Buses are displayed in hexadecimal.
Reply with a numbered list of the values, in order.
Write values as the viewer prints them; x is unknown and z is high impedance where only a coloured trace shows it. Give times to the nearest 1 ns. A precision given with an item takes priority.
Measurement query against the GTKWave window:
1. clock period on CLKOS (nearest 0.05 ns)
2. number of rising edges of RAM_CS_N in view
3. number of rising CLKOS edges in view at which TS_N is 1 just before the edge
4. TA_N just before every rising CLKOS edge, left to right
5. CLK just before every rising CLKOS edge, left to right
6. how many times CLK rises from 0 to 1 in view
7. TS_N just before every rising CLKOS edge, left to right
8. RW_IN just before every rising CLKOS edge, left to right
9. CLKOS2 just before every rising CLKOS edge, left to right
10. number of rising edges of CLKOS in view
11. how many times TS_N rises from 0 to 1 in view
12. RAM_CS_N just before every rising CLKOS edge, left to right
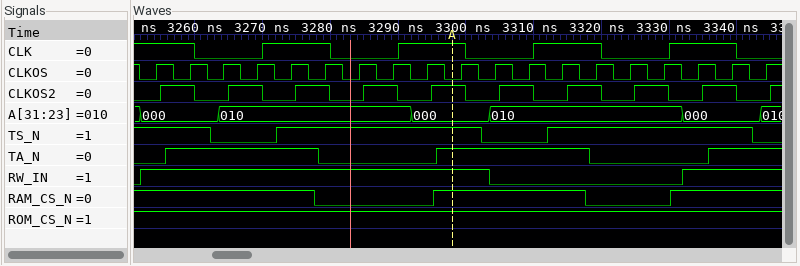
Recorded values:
1. 5 ns
2. 2
3. 14
4. 0 1 1 1 1 0 0 0 0 1 1 1 1 0 0 0 0 1 1
5. 1 1 0 0 1 1 0 0 1 1 0 0 1 1 0 0 1 1 0
6. 4
7. 1 1 0 0 1 1 1 1 1 1 0 0 1 1 1 1 1 1 0
8. 1 1 1 1 1 1 1 1 1 1 0 0 0 0 0 0 1 1 1
9. 0 1 0 1 0 1 0 1 0 1 0 1 0 1 0 1 0 1 0
10. 19
11. 2
12. 1 1 1 1 1 0 0 0 0 1 1 1 1 0 0 0 1 1 1
